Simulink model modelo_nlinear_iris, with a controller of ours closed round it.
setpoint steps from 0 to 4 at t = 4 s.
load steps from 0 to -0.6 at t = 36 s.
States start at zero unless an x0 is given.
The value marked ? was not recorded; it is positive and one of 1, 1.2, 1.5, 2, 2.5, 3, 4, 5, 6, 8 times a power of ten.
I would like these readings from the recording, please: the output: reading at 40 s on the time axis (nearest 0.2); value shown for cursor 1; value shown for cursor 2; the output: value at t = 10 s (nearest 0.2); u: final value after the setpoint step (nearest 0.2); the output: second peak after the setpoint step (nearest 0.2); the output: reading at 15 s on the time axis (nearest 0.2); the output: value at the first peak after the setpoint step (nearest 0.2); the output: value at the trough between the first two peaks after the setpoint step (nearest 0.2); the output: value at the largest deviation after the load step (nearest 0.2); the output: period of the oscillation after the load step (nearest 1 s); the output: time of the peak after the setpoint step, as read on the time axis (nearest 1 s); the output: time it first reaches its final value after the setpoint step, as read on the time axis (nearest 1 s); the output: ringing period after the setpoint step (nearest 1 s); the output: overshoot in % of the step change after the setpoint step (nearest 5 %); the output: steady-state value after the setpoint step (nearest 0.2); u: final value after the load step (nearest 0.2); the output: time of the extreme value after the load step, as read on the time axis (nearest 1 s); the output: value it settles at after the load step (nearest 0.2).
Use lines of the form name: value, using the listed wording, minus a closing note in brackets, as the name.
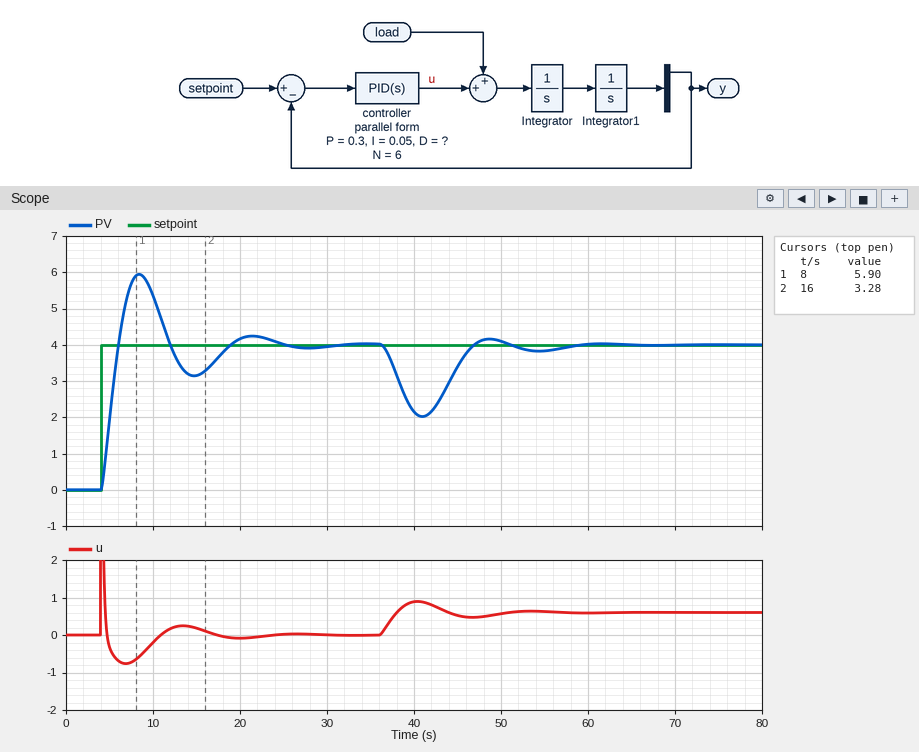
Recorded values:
the output: reading at 40 s on the time axis: 2.2
value shown for cursor 1: 5.90
value shown for cursor 2: 3.28
the output: value at t = 10 s: 5.4
u: final value after the setpoint step: 0.0
the output: second peak after the setpoint step: 4.2
the output: reading at 15 s on the time axis: 3.2
the output: value at the first peak after the setpoint step: 6.0
the output: value at the trough between the first two peaks after the setpoint step: 3.2
the output: value at the largest deviation after the load step: 2.0
the output: period of the oscillation after the load step: 13 s
the output: time of the peak after the setpoint step, as read on the time axis: 8 s
the output: time it first reaches its final value after the setpoint step, as read on the time axis: 6 s
the output: ringing period after the setpoint step: 13 s
the output: overshoot in % of the step change after the setpoint step: 50 %
the output: steady-state value after the setpoint step: 4.0
u: final value after the load step: 0.6
the output: time of the extreme value after the load step, as read on the time axis: 41 s
the output: value it settles at after the load step: 4.0
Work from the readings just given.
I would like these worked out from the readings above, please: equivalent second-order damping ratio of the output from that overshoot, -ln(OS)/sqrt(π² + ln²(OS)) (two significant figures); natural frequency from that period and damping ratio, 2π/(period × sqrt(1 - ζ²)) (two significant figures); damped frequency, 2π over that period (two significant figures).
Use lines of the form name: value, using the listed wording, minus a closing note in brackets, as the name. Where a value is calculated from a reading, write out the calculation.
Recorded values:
equivalent second-order damping ratio of the output from that overshoot, -ln(OS)/sqrt(π² + ln²(OS)): ln(0.5) = -0.693; 0.693 / sqrt(9.870 + 0.480) = 0.22
natural frequency from that period and damping ratio, 2π/(period × sqrt(1 - ζ²)): 2π / (13 × sqrt(1 - 0.22²)) = 0.50 rad/s
damped frequency, 2π over that period: 2π / 13 = 0.48 rad/s
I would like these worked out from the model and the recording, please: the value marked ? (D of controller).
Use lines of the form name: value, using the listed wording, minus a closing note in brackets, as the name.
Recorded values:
the value marked ?: 0.5
